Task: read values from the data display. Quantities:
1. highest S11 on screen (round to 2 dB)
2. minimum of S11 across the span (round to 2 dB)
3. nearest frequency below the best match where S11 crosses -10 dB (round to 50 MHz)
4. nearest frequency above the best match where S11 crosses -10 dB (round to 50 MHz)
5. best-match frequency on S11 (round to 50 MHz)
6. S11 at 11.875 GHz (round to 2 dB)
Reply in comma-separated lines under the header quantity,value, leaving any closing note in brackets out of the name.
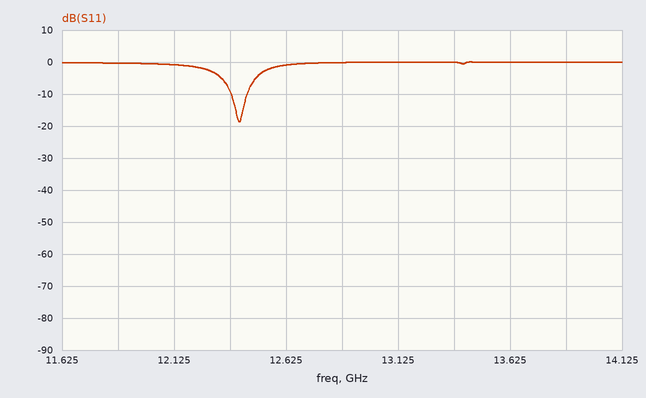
quantity,value
highest S11 on screen,0 dB
minimum of S11 across the span,-18 dB
nearest frequency below the best match where S11 crosses -10 dB,12.40 GHz
nearest frequency above the best match where S11 crosses -10 dB,12.45 GHz
best-match frequency on S11,12.40 GHz
S11 at 11.875 GHz,0 dB
